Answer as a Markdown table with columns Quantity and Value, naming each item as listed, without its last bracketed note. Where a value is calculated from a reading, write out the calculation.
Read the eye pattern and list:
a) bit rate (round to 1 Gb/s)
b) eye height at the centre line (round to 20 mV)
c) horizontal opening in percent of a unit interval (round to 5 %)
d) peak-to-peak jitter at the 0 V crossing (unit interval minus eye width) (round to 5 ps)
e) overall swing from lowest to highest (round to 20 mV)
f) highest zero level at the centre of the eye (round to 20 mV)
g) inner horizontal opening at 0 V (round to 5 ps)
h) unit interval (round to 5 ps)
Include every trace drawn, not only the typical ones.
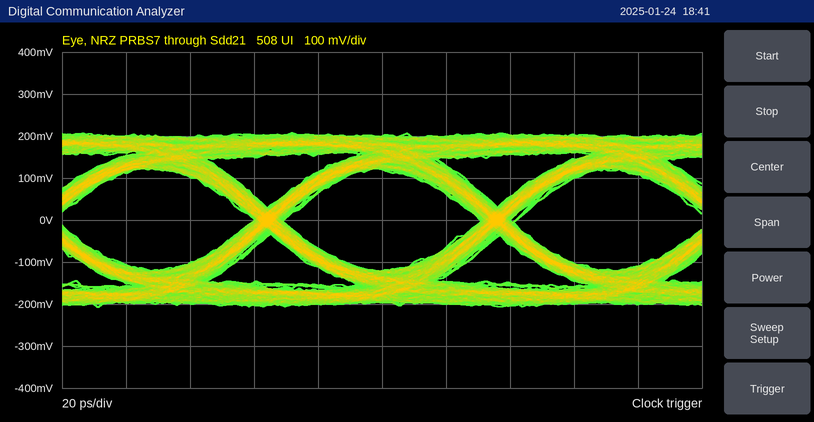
| Quantity | Value |
|---|---|
| bit rate | 14 Gb/s |
| eye height at the centre line | 240 mV |
| horizontal opening in percent of a unit interval | 60 ps / 70 ps ≈ 85.7 %, so 85 % to the nearest 5 % |
| peak-to-peak jitter at the 0 V crossing (unit interval minus eye width) | 10 ps |
| overall swing from lowest to highest | 420 mV |
| highest zero level at the centre of the eye | -120 mV |
| inner horizontal opening at 0 V | 60 ps |
| unit interval | 70 ps |
